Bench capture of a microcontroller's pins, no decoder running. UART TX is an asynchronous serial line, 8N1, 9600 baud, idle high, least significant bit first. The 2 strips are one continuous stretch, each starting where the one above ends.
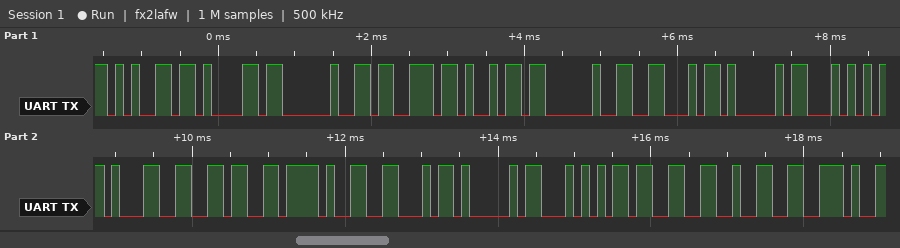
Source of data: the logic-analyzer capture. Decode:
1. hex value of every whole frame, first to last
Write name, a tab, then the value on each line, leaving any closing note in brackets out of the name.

hex value of every whole frame, first to last	0x65 0x61 0x20 0x73 0x69 0x20 0x46 0x41 0x54 0x31 0x36 0x2F 0x46 0x41 0x54 0x33 0x32 0x2E
